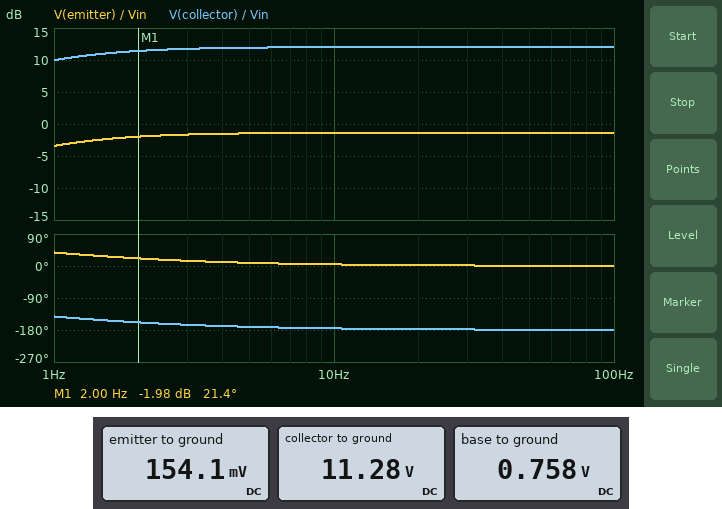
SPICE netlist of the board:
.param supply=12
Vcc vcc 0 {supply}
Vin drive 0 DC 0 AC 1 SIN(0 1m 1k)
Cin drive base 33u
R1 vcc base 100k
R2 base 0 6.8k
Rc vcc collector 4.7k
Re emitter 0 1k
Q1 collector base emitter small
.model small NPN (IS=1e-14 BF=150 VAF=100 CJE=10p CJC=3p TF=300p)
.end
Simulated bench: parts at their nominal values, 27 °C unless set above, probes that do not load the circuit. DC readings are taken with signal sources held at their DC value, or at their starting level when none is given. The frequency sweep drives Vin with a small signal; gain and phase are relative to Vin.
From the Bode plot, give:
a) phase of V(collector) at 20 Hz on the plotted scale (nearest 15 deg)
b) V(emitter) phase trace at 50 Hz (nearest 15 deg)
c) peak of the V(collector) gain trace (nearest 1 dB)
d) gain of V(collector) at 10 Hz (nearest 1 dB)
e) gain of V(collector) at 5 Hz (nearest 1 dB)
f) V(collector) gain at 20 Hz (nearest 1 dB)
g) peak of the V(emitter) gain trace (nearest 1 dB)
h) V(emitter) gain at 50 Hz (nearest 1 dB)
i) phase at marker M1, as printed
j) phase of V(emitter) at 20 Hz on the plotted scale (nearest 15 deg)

-180 deg
0 deg
12 dB
12 dB
12 dB
12 dB
-1 dB
-1 dB
21.4 deg
0 deg
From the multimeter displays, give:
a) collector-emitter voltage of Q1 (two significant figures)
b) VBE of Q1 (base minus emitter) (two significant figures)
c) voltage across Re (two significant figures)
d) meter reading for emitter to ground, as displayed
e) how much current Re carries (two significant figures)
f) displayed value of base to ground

11 V
600 mV
150 mV
154.1 mV
150 µA
0.758 V
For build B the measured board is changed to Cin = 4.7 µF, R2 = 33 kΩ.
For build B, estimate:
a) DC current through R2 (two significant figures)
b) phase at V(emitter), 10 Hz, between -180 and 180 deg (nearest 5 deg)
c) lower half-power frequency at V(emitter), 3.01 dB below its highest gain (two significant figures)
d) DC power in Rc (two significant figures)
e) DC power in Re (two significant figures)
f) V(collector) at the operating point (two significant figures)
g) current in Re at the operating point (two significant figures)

80 µA
10 deg
1.6 Hz
18 mW
3.9 mW
2.8 V
2.0 mA
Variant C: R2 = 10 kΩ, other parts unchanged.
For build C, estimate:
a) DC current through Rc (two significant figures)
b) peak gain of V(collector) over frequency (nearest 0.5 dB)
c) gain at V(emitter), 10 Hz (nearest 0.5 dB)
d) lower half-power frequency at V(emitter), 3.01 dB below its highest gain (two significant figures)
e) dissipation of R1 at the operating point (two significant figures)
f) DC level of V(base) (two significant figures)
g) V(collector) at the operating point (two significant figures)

430 µA
13.0 dB
-0.5 dB
560 mHz
1.2 mW
1.1 V
10 V
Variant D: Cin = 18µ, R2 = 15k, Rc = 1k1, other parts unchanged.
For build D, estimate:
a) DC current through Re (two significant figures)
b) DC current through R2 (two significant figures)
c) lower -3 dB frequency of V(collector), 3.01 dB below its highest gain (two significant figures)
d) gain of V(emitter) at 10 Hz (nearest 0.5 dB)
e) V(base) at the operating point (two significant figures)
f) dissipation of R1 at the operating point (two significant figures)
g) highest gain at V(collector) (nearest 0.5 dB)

850 µA
100 µA
730 mHz
-0.5 dB
1.5 V
1.1 mW
0.5 dB
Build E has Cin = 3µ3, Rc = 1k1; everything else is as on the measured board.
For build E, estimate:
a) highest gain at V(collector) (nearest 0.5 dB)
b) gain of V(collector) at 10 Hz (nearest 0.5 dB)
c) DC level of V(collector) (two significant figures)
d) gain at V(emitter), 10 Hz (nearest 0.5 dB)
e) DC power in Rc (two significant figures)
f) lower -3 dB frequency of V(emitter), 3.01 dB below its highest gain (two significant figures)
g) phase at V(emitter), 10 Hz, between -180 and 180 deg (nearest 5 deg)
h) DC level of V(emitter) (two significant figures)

-0.5 dB
-2.5 dB
12 V
-3.5 dB
26 µW
7.8 Hz
40 deg
150 mV
